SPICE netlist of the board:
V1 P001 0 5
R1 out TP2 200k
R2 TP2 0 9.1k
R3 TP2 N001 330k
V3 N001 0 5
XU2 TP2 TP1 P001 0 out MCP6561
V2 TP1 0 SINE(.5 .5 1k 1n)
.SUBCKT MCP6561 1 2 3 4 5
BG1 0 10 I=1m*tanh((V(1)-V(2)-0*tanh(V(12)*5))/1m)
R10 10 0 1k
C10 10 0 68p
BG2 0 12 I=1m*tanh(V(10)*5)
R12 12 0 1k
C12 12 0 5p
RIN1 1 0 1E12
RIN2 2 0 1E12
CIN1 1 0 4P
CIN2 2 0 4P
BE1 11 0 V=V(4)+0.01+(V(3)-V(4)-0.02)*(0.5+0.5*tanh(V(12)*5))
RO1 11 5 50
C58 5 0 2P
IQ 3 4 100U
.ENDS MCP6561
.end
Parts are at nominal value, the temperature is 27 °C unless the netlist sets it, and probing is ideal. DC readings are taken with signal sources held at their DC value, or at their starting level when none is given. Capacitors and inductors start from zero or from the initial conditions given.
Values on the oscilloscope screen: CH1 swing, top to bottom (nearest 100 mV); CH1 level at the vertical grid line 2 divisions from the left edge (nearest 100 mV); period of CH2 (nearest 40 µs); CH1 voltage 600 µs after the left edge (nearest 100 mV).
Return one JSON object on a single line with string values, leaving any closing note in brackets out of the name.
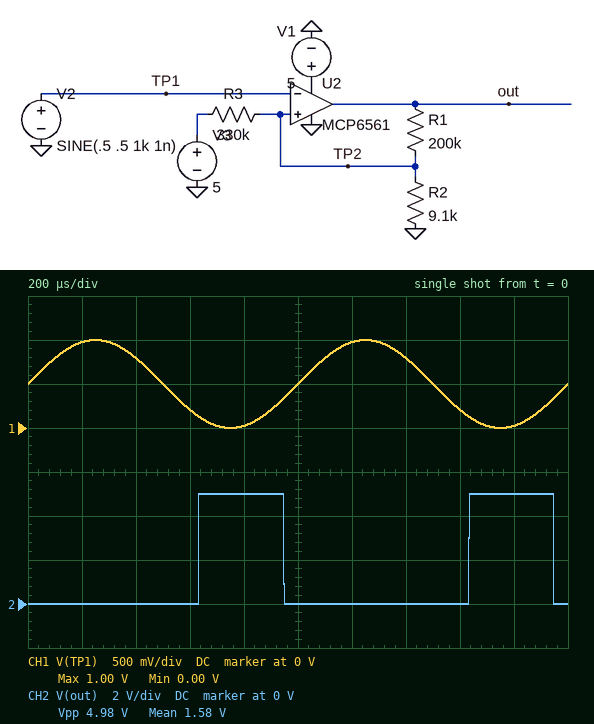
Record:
{"CH1 swing, top to bottom": "1.0 V", "CH1 level at the vertical grid line 2 divisions from the left edge": "800 mV", "period of CH2": "1.00 ms", "CH1 voltage 600 µs after the left edge": "200 mV"}
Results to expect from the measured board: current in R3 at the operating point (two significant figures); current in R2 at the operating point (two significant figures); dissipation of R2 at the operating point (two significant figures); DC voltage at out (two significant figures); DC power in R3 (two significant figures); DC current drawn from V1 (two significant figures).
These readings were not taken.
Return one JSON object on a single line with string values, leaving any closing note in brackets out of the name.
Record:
{"current in R3 at the operating point": "15 µA", "current in R2 at the operating point": "14 µA", "dissipation of R2 at the operating point": "1.8 µW", "DC voltage at out": "10 mV", "DC power in R3": "72 µW", "DC current drawn from V1": "100 µA"}
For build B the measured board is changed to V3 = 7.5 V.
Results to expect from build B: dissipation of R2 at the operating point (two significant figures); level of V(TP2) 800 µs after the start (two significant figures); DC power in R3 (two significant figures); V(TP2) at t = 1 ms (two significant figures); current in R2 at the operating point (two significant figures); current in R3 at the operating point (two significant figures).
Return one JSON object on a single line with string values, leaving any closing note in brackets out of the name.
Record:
{"dissipation of R2 at the operating point": "4.1 µW", "level of V(TP2) 800 µs after the start": "400 mV", "DC power in R3": "160 µW", "V(TP2) at t = 1 ms": "190 mV", "current in R2 at the operating point": "21 µA", "current in R3 at the operating point": "22 µA"}
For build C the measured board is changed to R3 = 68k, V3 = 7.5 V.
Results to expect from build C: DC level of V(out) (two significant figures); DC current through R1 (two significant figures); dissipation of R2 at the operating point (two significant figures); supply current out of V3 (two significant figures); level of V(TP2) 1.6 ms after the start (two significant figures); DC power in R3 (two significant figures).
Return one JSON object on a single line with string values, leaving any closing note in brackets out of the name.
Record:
{"DC level of V(out)": "5.0 V", "DC current through R1": "20 µA", "dissipation of R2 at the operating point": "120 µW", "supply current out of V3": "95 µA", "level of V(TP2) 1.6 ms after the start": "1.0 V", "DC power in R3": "610 µW"}
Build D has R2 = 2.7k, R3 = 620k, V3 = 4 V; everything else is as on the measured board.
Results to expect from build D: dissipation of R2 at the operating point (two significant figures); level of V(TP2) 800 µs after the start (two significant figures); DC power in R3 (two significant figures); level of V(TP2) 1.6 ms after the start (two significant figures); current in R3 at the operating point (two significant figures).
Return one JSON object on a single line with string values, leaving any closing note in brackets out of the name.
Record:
{"dissipation of R2 at the operating point": "110 nW", "level of V(TP2) 800 µs after the start": "83 mV", "DC power in R3": "26 µW", "level of V(TP2) 1.6 ms after the start": "17 mV", "current in R3 at the operating point": "6.4 µA"}
